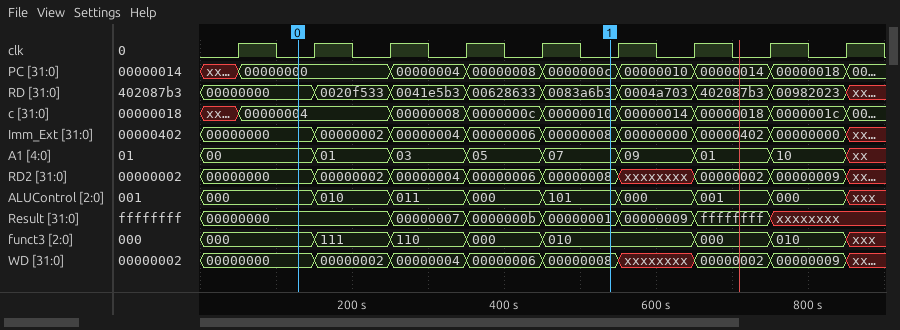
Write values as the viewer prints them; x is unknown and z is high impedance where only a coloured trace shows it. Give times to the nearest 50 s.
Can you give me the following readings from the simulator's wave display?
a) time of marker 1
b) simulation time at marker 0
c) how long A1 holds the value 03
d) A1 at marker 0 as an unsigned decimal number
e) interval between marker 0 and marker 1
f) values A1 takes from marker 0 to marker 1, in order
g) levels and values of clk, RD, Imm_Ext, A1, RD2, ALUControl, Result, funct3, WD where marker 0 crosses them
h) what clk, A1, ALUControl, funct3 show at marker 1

550 s
150 s
100 s
0
400 s
00, 01, 03, 05, 07
clk=0, RD=00000000, Imm_Ext=00000000, A1=00, RD2=00000000, ALUControl=000, Result=00000000, funct3=000, WD=00000000
clk=0, A1=07, ALUControl=101, funct3=010
